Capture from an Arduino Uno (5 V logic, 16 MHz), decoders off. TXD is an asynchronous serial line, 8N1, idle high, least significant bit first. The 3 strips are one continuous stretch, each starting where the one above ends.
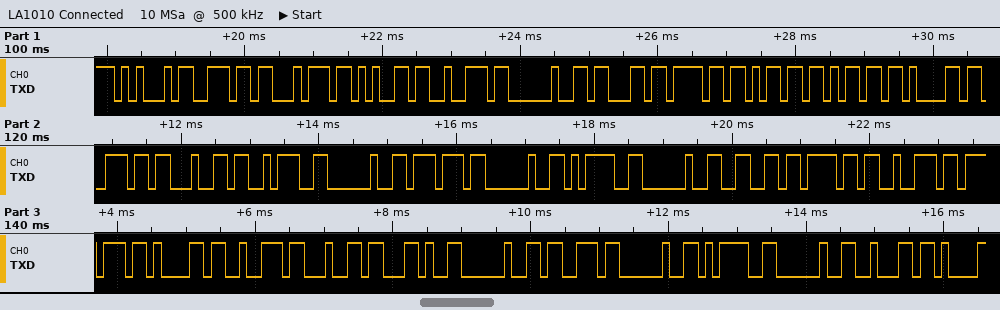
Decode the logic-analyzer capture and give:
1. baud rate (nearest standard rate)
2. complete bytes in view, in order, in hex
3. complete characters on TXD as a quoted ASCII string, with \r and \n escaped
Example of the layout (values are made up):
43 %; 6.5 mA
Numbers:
9600 baud; 45 6E 74 65 72 20 63 6F 6D 6D 61 6E 64 3A 20 77 20 3D 20 66 6F 72 77 61 72 64 2C 20 73 20 3D 20 62; "Enter command: w = forward, s = b"
